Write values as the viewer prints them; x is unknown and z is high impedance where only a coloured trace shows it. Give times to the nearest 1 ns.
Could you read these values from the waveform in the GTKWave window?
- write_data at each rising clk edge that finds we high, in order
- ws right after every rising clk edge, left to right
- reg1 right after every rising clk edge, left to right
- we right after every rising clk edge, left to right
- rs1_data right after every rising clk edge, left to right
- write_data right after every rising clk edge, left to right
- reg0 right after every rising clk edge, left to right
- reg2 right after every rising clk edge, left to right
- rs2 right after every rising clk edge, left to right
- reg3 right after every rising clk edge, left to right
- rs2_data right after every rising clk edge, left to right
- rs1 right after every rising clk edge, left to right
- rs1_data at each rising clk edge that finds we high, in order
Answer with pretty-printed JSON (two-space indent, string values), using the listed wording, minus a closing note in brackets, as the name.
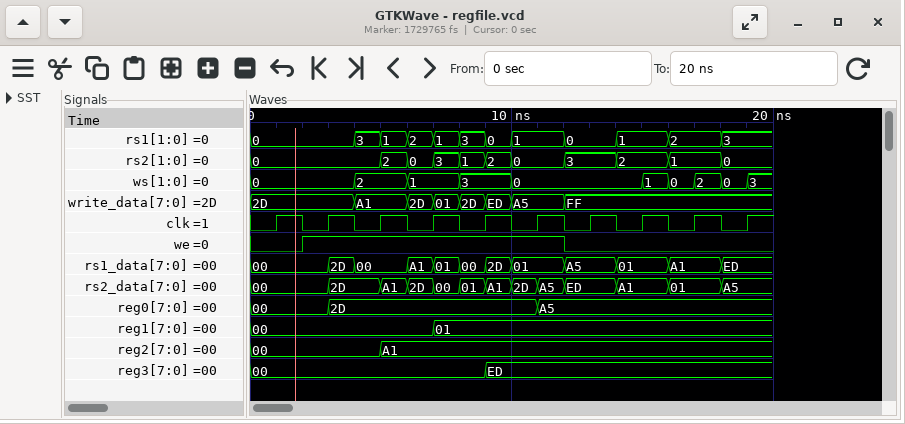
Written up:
{
  "write_data at each rising clk edge that finds we high, in order": "2D, A1, 2D, 2D, A5",
  "ws right after every rising clk edge, left to right": "0, 0, 2, 1, 3, 0, 0, 1, 2, 3",
  "reg1 right after every rising clk edge, left to right": "00, 00, 00, 01, 01, 01, 01, 01, 01, 01",
  "we right after every rising clk edge, left to right": "0 1 1 1 1 1 0 0 0 0",
  "rs1_data right after every rising clk edge, left to right": "00, 2D, 00, 01, 2D, 01, A5, 01, A1, ED",
  "write_data right after every rising clk edge, left to right": "2D, 2D, A1, 01, ED, A5, FF, FF, FF, FF",
  "reg0 right after every rising clk edge, left to right": "00, 2D, 2D, 2D, 2D, A5, A5, A5, A5, A5",
  "reg2 right after every rising clk edge, left to right": "00, 00, A1, A1, A1, A1, A1, A1, A1, A1",
  "rs2 right after every rising clk edge, left to right": "0, 0, 2, 3, 2, 0, 3, 2, 1, 0",
  "reg3 right after every rising clk edge, left to right": "00, 00, 00, 00, ED, ED, ED, ED, ED, ED",
  "rs2_data right after every rising clk edge, left to right": "00, 2D, A1, 00, A1, A5, ED, A1, 01, A5",
  "rs1 right after every rising clk edge, left to right": "0, 0, 1, 1, 0, 1, 0, 1, 2, 3",
  "rs1_data at each rising clk edge that finds we high, in order": "00, 00, A1, 00, 01"
}
